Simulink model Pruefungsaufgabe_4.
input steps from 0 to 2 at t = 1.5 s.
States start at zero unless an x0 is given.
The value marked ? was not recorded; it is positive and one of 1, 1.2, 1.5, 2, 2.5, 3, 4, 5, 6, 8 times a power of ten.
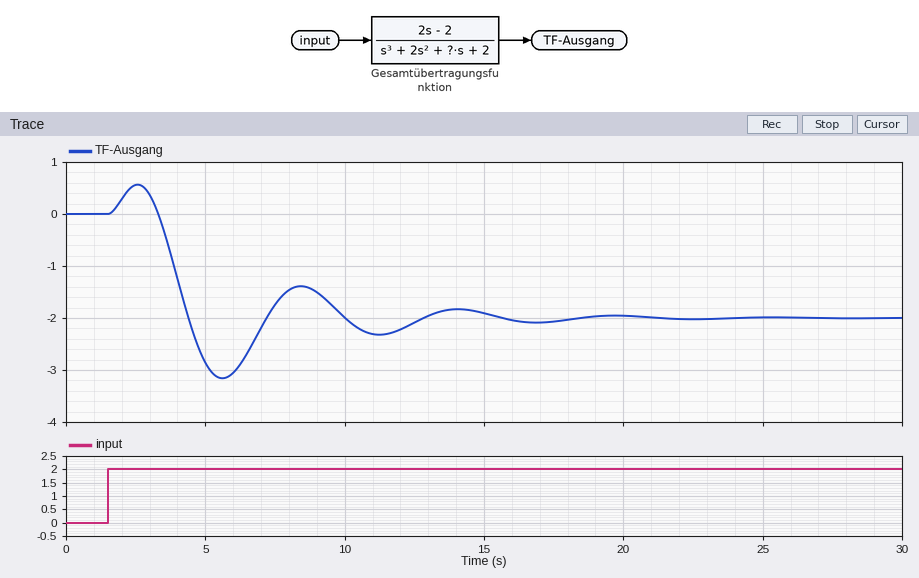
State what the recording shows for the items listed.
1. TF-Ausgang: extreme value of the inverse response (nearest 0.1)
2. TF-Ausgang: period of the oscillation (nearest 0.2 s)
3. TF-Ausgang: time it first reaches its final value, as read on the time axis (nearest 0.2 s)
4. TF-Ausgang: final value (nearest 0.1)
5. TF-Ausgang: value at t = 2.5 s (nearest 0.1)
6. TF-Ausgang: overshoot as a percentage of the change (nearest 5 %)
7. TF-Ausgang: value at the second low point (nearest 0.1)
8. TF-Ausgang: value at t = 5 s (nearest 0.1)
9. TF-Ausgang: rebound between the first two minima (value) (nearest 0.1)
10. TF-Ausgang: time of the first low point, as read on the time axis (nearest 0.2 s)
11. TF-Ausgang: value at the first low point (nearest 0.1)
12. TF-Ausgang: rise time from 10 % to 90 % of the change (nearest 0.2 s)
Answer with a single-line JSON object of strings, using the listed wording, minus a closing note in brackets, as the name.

{"TF-Ausgang: extreme value of the inverse response": "0.6", "TF-Ausgang: period of the oscillation": "5.6 s", "TF-Ausgang: time it first reaches its final value, as read on the time axis": "4.4 s", "TF-Ausgang: final value": "-2.0", "TF-Ausgang: value at t = 2.5 s": "0.6", "TF-Ausgang: overshoot as a percentage of the change": "60 %", "TF-Ausgang: value at the second low point": "-2.3", "TF-Ausgang: value at t = 5 s": "-2.9", "TF-Ausgang: rebound between the first two minima (value)": "-1.4", "TF-Ausgang: time of the first low point, as read on the time axis": "5.6 s", "TF-Ausgang: value at the first low point": "-3.2", "TF-Ausgang: rise time from 10 % to 90 % of the change": "0.8 s"}
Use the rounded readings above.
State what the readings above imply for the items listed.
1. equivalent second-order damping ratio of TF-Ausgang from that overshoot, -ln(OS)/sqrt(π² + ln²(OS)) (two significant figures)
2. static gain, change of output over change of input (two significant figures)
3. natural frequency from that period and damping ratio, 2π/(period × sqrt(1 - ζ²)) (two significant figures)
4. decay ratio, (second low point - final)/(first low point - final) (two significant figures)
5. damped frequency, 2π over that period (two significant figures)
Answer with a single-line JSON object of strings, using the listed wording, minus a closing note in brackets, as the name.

{"equivalent second-order damping ratio of TF-Ausgang from that overshoot, -ln(OS)/sqrt(π² + ln²(OS))": "0.16", "static gain, change of output over change of input": "-1.0", "natural frequency from that period and damping ratio, 2π/(period × sqrt(1 - ζ²))": "1.1 rad/s", "decay ratio, (second low point - final)/(first low point - final)": "0.25", "damped frequency, 2π over that period": "1.1 rad/s"}
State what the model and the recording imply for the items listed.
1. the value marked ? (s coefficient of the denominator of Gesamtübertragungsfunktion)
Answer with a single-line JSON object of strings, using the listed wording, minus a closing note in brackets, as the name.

{"the value marked ?": "2"}
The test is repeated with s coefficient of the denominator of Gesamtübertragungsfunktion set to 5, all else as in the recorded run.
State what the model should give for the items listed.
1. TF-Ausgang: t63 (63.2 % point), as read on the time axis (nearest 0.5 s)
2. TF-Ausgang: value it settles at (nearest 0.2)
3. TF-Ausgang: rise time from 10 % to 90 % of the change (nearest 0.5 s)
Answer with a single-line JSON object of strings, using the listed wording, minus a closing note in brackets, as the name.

{"TF-Ausgang: t63 (63.2 % point), as read on the time axis": "4.5 s", "TF-Ausgang: value it settles at": "-2.0", "TF-Ausgang: rise time from 10 % to 90 % of the change": "4.0 s"}
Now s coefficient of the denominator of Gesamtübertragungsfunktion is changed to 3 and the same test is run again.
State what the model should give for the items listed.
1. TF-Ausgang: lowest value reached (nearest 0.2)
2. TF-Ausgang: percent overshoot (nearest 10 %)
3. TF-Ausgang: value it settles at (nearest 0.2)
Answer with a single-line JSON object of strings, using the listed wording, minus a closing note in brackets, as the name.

{"TF-Ausgang: lowest value reached": "-2.4", "TF-Ausgang: percent overshoot": "20 %", "TF-Ausgang: value it settles at": "-2.0"}
